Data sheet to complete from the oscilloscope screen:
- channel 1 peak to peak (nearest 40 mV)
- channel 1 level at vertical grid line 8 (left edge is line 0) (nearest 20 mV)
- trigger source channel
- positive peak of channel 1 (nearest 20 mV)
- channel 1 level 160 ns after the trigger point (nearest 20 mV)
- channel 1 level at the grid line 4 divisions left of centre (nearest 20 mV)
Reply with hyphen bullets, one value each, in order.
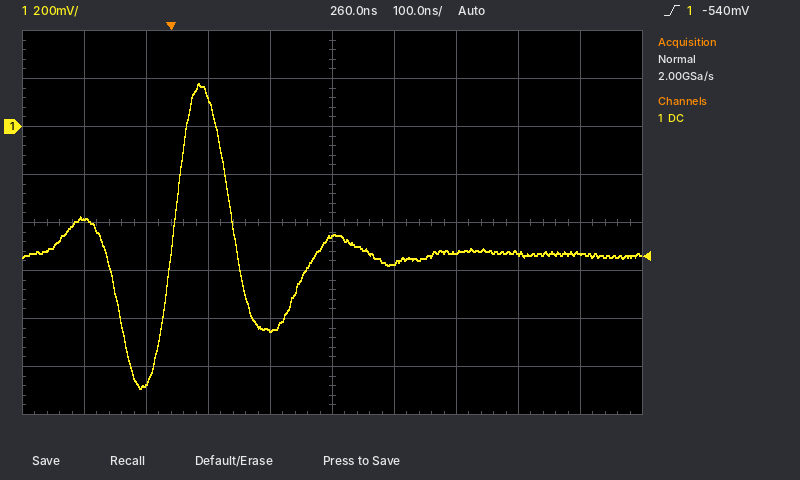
- 1.28 V
- -520 mV
- channel 1
- 180 mV
- -840 mV
- -380 mV
